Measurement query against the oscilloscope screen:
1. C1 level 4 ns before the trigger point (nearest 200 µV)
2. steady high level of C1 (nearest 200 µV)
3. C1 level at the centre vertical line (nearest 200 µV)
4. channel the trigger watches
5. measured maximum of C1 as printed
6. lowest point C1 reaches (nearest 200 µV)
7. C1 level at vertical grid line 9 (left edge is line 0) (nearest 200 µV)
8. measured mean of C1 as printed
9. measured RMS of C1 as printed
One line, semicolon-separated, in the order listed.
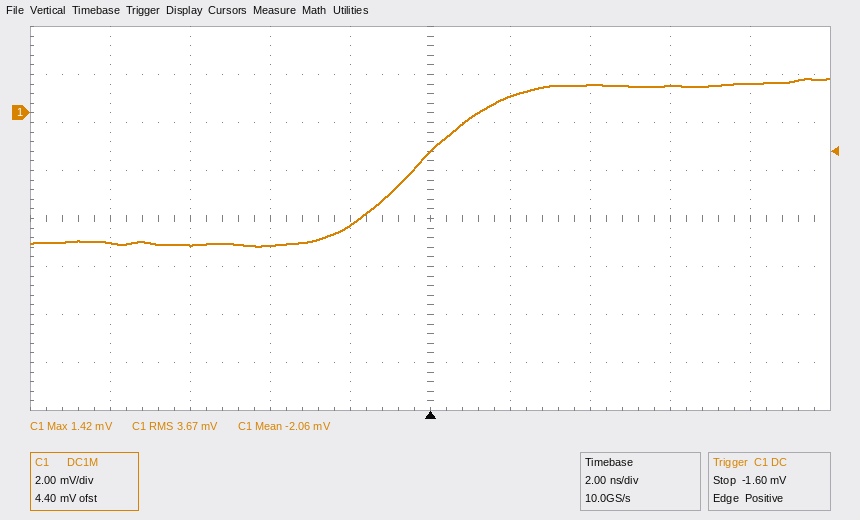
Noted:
-5.6 mV; 1.2 mV; -1.6 mV; C1; 1.42 mV; -5.6 mV; 1.2 mV; -2.06 mV; 3.67 mV
